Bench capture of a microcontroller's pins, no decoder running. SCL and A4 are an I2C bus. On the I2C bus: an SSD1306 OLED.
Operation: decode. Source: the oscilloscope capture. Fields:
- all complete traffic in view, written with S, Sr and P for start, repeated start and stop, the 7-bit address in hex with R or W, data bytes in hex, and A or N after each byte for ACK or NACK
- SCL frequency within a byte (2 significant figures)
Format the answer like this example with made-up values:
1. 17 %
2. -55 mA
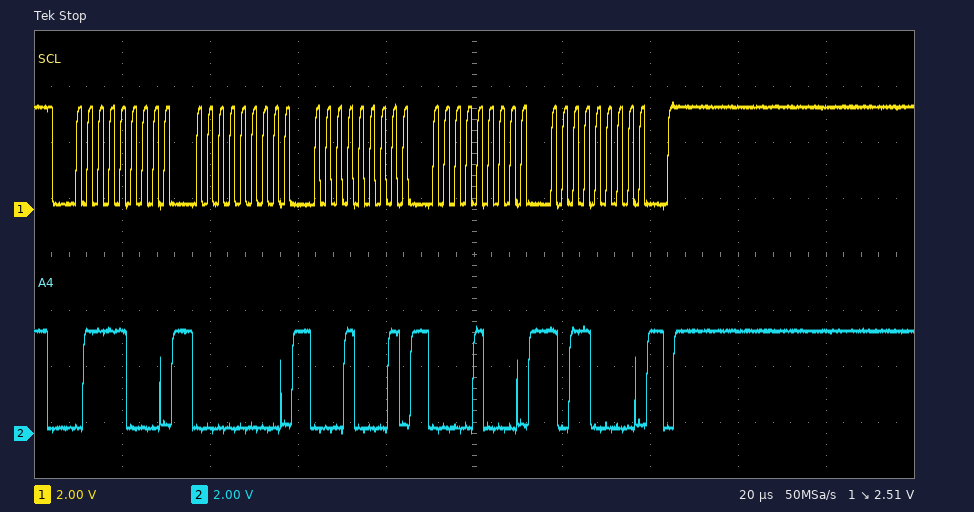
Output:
1. S 3CW A 00 A 11 A 08 A B0 A P
2. 400 kHz
